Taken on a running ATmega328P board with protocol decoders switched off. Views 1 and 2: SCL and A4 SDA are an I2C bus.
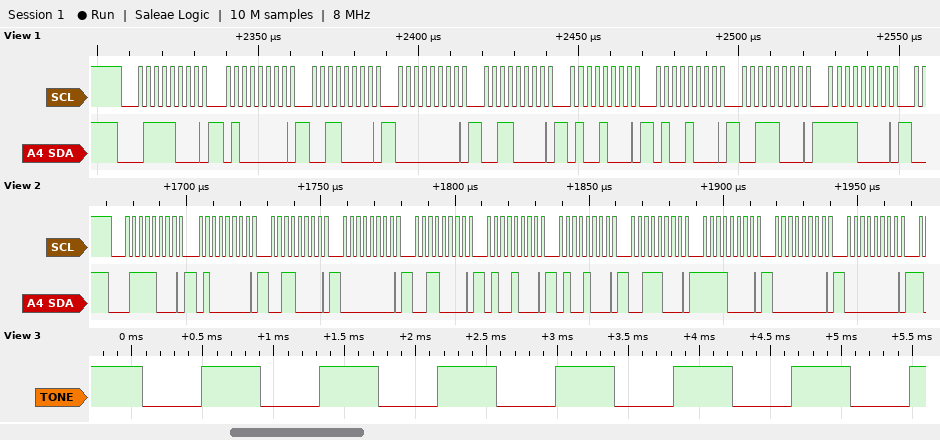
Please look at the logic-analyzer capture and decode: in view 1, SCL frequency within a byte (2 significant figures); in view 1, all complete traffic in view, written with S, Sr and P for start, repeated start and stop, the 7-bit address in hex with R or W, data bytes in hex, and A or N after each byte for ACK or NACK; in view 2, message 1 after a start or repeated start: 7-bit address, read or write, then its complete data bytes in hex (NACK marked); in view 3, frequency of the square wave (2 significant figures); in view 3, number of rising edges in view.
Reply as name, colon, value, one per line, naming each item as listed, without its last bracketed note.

in view 1, SCL frequency within a byte: 400 kHz
in view 1, all complete traffic in view, written with S, Sr and P for start, repeated start and stop, the 7-bit address in hex with R or W, data bytes in hex, and A or N after each byte for ACK or NACK: S 3CW A 40 A 30 A 00 A 30 A 48 A 48 A 38 A F0 A
in view 2, message 1 after a start or repeated start: 7-bit address, read or write, then its complete data bytes in hex: 0x3C write: 40 30 00 30 48 48 38 F0 00 00
in view 3, frequency of the square wave: 1.2 kHz
in view 3, number of rising edges in view: 7
